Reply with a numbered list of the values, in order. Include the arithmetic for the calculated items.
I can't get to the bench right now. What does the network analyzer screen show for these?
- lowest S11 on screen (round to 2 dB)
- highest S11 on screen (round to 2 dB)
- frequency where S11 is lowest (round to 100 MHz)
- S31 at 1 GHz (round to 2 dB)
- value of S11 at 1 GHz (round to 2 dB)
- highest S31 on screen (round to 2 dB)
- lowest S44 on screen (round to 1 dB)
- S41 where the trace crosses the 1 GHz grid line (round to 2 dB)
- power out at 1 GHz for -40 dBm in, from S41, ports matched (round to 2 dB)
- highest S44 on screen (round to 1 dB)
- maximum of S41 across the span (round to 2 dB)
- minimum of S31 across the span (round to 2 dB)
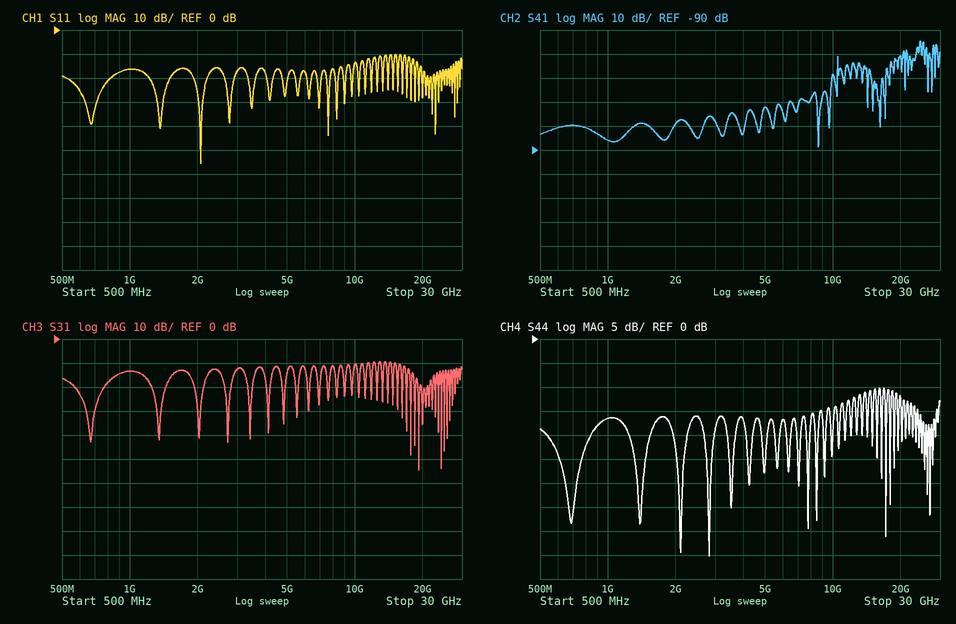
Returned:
1. -56 dB
2. -10 dB
3. 2.1 GHz
4. -14 dB
5. -16 dB
6. -10 dB
7. -45 dB
8. -86 dB
9. -40 dBm + (-86 dB) = -126 dBm
10. -10 dB
11. -44 dB
12. -54 dB
